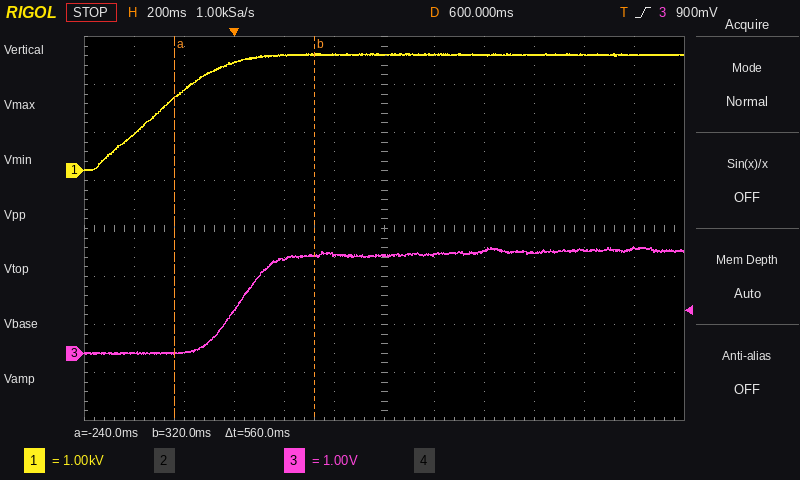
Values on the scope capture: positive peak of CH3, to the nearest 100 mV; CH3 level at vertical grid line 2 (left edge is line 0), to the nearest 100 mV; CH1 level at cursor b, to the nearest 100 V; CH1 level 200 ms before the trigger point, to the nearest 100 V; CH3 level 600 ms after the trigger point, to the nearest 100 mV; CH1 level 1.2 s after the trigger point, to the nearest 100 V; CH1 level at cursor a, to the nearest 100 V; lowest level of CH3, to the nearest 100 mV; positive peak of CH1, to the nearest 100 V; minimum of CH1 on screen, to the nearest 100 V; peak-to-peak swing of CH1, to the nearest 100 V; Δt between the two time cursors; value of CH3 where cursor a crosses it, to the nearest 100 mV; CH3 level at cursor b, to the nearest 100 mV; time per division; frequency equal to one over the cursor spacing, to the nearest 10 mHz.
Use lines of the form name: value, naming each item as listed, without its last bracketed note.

positive peak of CH3, to the nearest 100 mV: 2.2 V
CH3 level at vertical grid line 2 (left edge is line 0), to the nearest 100 mV: 0.0 V
CH1 level at cursor b, to the nearest 100 V: 2.4 kV
CH1 level 200 ms before the trigger point, to the nearest 100 V: 1.7 kV
CH3 level 600 ms after the trigger point, to the nearest 100 mV: 2.0 V
CH1 level 1.2 s after the trigger point, to the nearest 100 V: 2.4 kV
CH1 level at cursor a, to the nearest 100 V: 1.5 kV
lowest level of CH3, to the nearest 100 mV: 0.0 V
positive peak of CH1, to the nearest 100 V: 2.4 kV
minimum of CH1 on screen, to the nearest 100 V: 0.0 kV
peak-to-peak swing of CH1, to the nearest 100 V: 2.4 kV
Δt between the two time cursors: 560 ms
value of CH3 where cursor a crosses it, to the nearest 100 mV: 0.0 V
CH3 level at cursor b, to the nearest 100 mV: 2.0 V
time per division: 200 ms
frequency equal to one over the cursor spacing, to the nearest 10 mHz: 1.79 Hz
